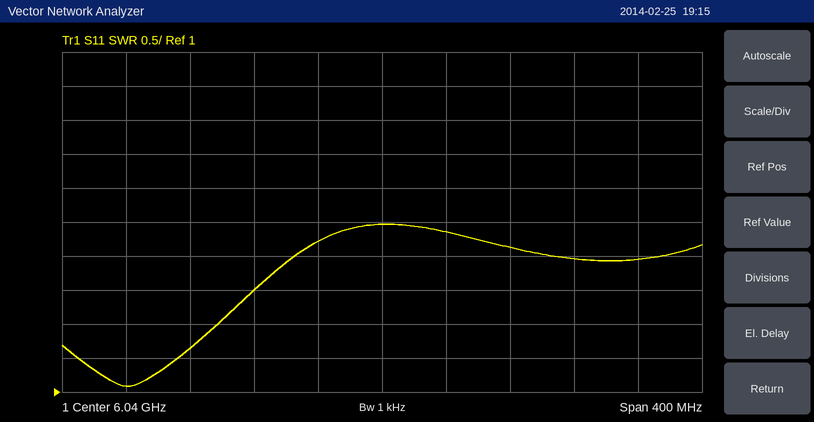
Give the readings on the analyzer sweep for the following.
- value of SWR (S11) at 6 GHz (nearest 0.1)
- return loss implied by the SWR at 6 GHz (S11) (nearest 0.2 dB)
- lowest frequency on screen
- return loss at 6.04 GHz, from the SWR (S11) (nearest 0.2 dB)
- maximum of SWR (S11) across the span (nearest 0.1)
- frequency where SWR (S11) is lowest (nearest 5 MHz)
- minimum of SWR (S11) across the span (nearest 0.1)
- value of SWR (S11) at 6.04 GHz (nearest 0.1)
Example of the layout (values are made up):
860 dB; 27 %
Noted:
3.2; 5.6 dB; 5.84 GHz; 5.2 dB; 3.5; 5.880 GHz; 1.1; 3.5
